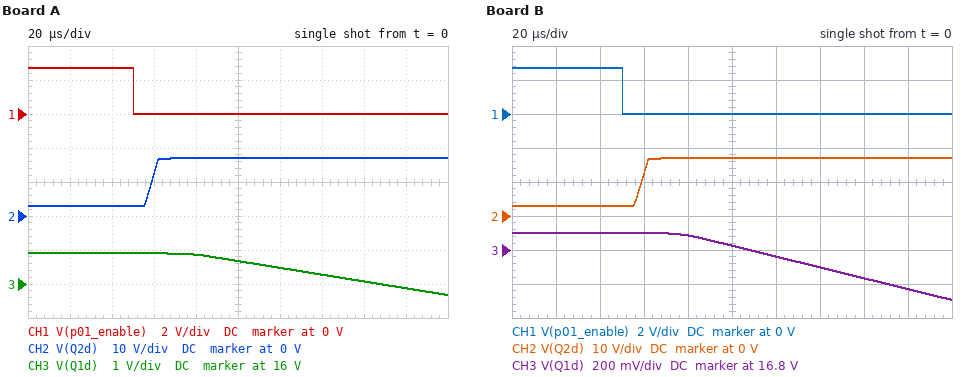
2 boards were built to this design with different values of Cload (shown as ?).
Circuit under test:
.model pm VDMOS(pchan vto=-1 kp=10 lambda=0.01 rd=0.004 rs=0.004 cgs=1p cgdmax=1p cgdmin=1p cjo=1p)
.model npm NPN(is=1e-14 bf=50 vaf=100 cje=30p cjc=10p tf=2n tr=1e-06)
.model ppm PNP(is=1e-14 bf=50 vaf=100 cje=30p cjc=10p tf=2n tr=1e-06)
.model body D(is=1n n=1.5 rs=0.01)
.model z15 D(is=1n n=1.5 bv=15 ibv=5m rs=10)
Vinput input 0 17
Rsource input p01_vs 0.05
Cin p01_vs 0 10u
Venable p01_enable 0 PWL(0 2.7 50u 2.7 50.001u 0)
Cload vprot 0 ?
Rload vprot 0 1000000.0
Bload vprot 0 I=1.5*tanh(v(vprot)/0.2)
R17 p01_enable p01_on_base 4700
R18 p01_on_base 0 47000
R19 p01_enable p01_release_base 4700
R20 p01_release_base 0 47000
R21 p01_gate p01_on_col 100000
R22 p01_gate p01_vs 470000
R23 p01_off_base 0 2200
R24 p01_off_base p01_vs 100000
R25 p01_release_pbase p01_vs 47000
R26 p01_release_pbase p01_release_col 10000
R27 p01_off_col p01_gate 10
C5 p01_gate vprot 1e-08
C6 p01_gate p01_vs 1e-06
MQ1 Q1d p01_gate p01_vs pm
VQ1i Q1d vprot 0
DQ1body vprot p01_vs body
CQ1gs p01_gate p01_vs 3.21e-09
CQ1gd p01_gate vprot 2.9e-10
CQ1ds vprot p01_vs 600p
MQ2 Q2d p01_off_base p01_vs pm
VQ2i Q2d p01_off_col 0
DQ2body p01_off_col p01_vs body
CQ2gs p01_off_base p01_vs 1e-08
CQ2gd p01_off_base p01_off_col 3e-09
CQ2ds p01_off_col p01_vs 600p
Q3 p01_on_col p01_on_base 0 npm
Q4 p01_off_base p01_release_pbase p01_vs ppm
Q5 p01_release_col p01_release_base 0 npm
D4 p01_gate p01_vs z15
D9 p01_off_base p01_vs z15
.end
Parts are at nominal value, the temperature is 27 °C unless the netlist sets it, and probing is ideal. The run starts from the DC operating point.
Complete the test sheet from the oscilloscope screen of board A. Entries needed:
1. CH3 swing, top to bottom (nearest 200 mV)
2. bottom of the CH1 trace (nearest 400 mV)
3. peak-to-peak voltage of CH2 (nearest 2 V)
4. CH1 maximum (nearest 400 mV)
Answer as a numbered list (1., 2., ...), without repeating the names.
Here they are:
1. 1.2 V
2. 0 V
3. 14 V
4. 2.8 V
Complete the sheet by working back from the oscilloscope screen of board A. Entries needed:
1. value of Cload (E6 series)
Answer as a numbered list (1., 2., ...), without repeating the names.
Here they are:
1. 150 µF
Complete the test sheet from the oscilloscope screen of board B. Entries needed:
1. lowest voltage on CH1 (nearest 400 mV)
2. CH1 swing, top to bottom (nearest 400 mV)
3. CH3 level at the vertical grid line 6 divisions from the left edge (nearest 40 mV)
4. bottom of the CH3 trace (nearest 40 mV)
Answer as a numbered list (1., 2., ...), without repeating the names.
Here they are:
1. 0 V
2. 2.8 V
3. 16.76 V
4. 16.52 V
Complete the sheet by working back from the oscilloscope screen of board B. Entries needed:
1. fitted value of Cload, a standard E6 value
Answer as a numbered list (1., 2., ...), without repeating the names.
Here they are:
1. 470 µF
